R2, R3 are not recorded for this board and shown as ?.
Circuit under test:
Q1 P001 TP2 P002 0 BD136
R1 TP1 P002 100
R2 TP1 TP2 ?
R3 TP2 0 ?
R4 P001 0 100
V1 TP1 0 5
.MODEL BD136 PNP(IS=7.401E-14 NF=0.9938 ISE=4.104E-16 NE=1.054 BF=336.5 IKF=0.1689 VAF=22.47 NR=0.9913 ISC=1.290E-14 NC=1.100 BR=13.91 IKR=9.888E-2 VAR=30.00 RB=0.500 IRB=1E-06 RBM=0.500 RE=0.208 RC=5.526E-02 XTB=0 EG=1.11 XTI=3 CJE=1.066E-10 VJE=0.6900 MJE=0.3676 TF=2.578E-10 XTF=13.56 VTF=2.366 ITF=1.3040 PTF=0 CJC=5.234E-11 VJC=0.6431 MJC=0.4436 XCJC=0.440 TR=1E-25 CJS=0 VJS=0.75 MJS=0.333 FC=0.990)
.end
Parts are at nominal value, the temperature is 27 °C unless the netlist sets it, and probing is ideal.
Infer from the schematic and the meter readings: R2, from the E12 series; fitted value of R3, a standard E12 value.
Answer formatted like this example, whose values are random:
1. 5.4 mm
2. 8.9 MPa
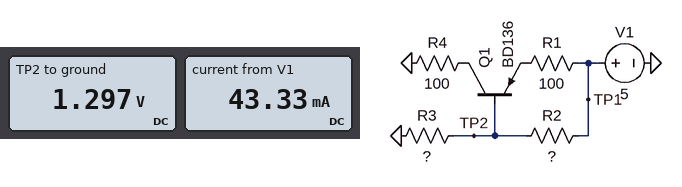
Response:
1. 270 Ω
2. 56 Ω
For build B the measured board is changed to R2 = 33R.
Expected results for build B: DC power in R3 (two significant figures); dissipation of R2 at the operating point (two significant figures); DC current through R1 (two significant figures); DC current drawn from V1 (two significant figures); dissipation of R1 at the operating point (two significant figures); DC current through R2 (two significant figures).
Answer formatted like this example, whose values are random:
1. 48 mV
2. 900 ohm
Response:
1. 180 mW
2. 100 mW
3. 12 mA
4. 68 mA
5. 14 mW
6. 56 mA
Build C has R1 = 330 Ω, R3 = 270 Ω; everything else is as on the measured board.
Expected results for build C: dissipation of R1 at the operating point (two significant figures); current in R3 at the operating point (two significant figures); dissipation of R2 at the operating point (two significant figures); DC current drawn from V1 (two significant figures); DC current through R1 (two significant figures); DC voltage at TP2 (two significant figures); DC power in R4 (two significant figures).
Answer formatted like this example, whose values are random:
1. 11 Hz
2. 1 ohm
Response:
1. 10 mW
2. 9.3 mA
3. 23 mW
4. 15 mA
5. 5.6 mA
6. 2.5 V
7. 3.1 mW
